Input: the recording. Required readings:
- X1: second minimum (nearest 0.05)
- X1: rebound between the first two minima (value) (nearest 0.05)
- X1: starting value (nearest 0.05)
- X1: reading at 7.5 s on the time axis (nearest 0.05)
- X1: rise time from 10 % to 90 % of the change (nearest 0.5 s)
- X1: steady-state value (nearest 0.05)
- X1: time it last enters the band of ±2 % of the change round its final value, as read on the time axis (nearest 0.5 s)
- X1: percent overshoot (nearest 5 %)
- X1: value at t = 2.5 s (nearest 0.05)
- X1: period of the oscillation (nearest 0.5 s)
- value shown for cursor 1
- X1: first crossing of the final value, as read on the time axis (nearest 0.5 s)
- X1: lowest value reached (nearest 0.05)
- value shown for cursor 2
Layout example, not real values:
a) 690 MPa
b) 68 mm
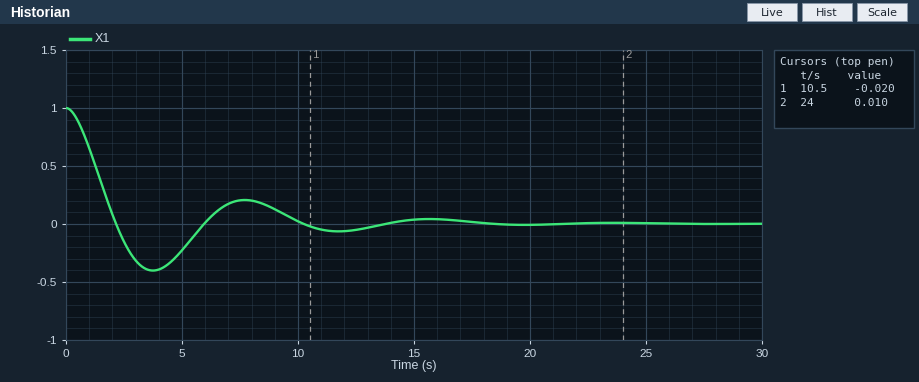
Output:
a) -0.05
b) 0.20
c) 1.00
d) 0.20
e) 1.5 s
f) 0.00
g) 17.5 s
h) 40 %
i) -0.15
j) 8.0 s
k) -0.020
l) 2.0 s
m) -0.40
n) 0.010
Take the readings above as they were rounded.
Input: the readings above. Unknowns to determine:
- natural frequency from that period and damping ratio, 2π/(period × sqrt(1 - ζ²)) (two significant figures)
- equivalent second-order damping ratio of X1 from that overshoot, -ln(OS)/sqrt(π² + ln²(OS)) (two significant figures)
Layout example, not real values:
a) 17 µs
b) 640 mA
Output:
a) 0.82 rad/s
b) 0.28
